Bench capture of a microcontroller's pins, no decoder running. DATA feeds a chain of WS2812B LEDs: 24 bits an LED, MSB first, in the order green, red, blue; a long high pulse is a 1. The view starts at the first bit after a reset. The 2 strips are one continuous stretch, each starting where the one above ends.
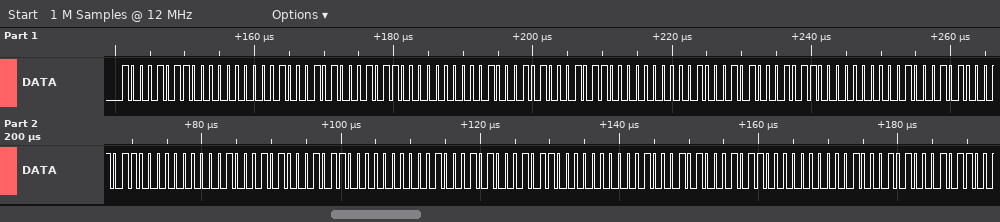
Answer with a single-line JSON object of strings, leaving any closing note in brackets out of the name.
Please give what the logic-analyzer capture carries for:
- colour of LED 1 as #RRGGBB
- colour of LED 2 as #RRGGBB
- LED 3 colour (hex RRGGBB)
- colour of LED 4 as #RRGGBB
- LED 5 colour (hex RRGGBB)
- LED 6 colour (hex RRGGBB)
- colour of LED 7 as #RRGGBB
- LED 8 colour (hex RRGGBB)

{"colour of LED 1 as #RRGGBB": "#008B22", "colour of LED 2 as #RRGGBB": "#008B22", "LED 3 colour": "#008B22", "colour of LED 4 as #RRGGBB": "#008B22", "LED 5 colour": "#008B22", "LED 6 colour": "#008B22", "colour of LED 7 as #RRGGBB": "#008B22", "LED 8 colour": "#008B22"}
